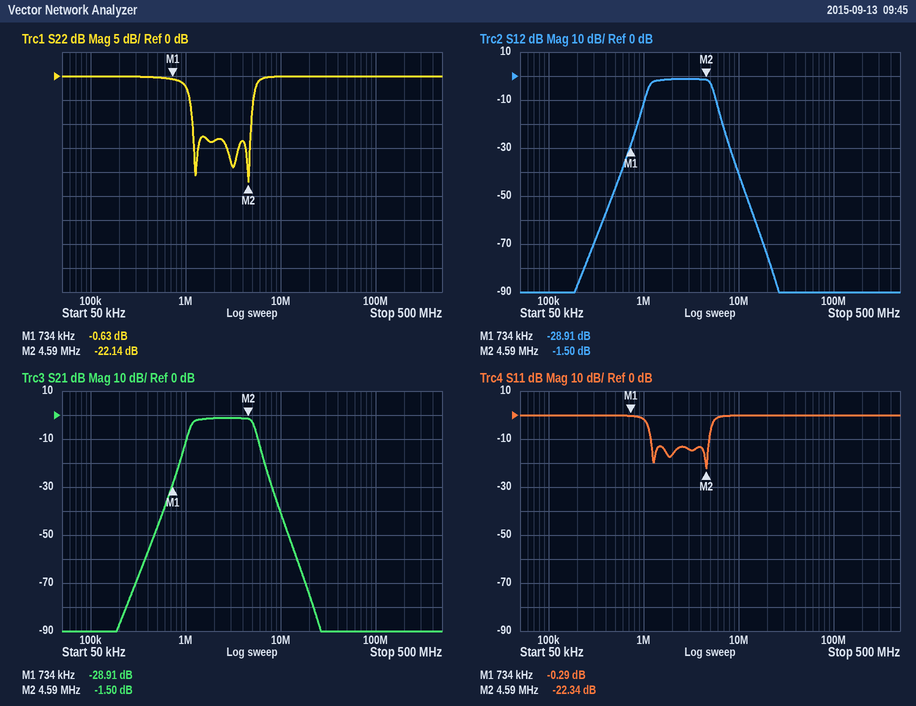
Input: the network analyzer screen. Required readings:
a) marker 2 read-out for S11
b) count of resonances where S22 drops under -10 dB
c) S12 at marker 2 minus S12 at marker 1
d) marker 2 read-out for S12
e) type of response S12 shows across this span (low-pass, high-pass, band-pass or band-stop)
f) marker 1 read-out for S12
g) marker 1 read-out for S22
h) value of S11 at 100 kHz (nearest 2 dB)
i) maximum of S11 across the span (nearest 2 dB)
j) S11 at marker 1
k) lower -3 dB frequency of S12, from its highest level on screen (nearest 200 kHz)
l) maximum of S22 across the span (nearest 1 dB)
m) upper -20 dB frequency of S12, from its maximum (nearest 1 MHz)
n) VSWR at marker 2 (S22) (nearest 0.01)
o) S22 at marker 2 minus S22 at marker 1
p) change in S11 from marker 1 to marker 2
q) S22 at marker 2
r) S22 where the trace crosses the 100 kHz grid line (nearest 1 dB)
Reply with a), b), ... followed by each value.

a) -22.34 dB
b) 3
c) 27.41 dB
d) -1.50 dB
e) band-pass
f) -28.91 dB
g) -0.63 dB
h) 0 dB
i) 0 dB
j) -0.29 dB
k) 1.2 MHz
l) 0 dB
m) 7 MHz
n) 1.17
o) -21.51 dB
p) -22.05 dB
q) -22.14 dB
r) 0 dB
